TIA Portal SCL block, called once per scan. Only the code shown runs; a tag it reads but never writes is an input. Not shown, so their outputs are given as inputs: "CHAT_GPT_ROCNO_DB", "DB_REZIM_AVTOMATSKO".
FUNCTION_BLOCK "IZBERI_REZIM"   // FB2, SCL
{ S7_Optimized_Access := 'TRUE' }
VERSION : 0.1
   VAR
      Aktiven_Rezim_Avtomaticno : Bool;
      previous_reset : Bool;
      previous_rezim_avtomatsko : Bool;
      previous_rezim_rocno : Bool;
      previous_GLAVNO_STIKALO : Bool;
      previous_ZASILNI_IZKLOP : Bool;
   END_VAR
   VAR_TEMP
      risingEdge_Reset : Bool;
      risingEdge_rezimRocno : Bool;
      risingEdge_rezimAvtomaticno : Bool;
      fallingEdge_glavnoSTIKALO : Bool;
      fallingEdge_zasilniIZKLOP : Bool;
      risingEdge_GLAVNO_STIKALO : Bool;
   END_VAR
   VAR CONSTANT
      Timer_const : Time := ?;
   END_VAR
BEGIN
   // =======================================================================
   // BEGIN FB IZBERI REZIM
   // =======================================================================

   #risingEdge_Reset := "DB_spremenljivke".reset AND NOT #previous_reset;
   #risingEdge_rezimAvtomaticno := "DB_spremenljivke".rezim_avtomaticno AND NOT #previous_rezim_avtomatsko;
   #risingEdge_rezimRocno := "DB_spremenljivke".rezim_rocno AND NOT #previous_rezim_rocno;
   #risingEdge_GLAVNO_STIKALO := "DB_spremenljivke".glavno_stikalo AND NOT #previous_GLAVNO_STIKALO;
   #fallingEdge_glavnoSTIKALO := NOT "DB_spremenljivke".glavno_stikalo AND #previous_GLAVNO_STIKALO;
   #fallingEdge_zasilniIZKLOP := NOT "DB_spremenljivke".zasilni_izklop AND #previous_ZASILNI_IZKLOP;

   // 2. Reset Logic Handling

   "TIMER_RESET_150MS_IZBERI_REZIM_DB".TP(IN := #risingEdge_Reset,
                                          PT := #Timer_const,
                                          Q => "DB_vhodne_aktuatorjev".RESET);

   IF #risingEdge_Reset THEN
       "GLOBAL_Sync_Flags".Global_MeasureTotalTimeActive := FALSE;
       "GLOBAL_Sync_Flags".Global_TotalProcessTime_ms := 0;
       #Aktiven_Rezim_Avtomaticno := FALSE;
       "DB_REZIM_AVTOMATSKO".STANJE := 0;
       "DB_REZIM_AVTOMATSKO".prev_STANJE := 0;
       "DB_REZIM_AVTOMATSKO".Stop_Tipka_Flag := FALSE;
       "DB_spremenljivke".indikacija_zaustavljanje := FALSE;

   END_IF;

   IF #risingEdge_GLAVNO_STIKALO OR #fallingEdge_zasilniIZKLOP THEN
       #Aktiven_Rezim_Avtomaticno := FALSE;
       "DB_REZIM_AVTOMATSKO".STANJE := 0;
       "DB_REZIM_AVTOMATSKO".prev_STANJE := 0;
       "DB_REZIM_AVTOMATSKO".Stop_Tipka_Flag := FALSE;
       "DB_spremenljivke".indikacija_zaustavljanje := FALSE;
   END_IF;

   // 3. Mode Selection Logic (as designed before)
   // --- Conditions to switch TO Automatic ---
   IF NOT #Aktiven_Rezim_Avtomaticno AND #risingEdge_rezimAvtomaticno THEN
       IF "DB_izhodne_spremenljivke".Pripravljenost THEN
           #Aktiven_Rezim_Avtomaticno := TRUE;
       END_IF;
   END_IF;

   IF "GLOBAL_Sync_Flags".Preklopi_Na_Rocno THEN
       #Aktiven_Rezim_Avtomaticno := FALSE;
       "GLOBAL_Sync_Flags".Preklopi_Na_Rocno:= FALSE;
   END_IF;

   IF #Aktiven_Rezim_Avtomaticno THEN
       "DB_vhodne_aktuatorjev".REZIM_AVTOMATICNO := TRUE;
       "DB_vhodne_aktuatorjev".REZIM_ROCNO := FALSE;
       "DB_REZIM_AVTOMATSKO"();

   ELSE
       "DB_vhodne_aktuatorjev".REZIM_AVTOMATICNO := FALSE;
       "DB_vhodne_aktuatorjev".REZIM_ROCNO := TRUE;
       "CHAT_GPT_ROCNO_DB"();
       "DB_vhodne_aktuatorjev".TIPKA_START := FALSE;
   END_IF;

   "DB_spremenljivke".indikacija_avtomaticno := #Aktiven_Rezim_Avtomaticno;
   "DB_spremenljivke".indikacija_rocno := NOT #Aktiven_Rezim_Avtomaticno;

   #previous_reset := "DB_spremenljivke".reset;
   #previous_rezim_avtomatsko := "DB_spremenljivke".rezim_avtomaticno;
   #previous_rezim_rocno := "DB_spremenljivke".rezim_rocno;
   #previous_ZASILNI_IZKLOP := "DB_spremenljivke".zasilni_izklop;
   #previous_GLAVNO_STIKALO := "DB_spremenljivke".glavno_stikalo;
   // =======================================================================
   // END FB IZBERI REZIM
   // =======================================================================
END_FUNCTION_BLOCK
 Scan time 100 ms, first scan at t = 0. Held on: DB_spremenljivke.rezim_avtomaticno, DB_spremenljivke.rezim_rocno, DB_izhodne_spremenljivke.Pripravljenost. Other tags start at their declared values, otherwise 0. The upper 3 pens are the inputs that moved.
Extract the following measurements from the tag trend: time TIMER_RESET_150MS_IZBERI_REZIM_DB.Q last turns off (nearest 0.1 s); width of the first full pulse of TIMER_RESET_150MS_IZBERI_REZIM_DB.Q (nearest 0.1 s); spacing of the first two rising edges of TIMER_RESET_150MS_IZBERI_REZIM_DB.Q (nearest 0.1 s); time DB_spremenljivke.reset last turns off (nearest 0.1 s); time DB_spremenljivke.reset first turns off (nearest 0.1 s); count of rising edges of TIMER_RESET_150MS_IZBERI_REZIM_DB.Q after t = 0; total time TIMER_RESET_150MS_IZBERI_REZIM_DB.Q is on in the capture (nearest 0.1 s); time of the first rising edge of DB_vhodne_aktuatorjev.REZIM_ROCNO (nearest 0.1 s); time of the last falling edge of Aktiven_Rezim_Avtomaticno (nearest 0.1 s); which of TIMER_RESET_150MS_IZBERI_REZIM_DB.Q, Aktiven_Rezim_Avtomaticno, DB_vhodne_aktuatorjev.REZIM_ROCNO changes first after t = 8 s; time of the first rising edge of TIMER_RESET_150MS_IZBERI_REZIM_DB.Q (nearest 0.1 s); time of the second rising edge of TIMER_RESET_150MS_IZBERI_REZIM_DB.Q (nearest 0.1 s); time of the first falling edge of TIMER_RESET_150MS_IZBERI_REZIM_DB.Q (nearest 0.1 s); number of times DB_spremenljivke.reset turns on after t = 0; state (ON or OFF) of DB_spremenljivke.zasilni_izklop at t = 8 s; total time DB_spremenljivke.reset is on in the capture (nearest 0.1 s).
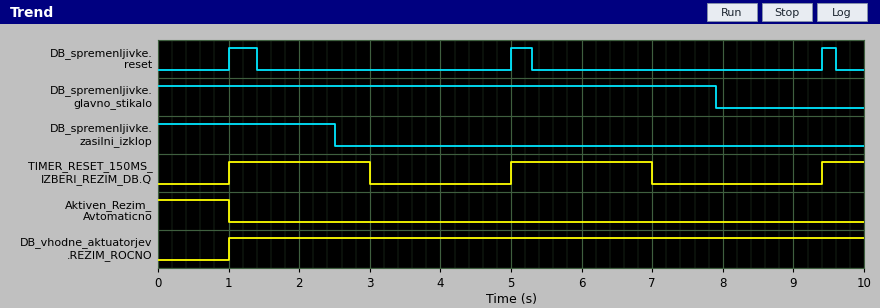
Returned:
7.0 s
2.0 s
4.0 s
9.6 s
1.4 s
3
4.6 s
1.0 s
1.0 s
TIMER_RESET_150MS_IZBERI_REZIM_DB.Q
1.0 s
5.0 s
3.0 s
3
OFF
0.9 s
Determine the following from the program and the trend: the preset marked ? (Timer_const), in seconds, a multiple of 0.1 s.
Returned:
2.0 s
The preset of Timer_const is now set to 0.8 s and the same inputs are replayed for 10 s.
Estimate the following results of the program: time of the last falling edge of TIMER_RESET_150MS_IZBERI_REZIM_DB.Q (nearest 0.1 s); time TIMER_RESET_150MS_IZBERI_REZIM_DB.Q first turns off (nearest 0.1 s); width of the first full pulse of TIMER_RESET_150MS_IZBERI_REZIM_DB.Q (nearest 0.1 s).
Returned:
5.8 s
1.8 s
0.8 s
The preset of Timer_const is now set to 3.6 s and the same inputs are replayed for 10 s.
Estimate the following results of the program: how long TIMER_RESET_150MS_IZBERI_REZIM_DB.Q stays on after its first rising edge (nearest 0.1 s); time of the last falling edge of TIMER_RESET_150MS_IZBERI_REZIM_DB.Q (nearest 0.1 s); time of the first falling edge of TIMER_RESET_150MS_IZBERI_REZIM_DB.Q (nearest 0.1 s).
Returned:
3.6 s
8.6 s
4.6 s
